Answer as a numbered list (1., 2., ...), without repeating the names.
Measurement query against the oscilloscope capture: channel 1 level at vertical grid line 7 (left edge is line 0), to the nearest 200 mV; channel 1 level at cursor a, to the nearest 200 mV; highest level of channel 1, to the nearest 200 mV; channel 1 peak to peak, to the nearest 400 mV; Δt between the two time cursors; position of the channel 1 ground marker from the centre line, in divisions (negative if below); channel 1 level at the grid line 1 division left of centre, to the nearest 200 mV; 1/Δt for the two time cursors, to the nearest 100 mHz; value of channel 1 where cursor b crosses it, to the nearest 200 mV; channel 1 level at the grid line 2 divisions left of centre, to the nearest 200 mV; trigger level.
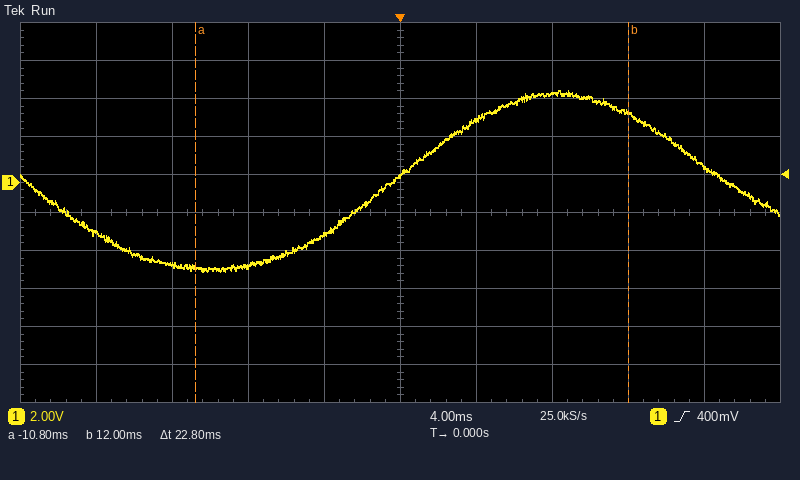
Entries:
1. 4.6 V
2. -4.4 V
3. 4.8 V
4. 9.6 V
5. 22.8 ms
6. +0.8 div
7. -2.8 V
8. 43.9 Hz
9. 3.6 V
10. -4.4 V
11. 400 mV
